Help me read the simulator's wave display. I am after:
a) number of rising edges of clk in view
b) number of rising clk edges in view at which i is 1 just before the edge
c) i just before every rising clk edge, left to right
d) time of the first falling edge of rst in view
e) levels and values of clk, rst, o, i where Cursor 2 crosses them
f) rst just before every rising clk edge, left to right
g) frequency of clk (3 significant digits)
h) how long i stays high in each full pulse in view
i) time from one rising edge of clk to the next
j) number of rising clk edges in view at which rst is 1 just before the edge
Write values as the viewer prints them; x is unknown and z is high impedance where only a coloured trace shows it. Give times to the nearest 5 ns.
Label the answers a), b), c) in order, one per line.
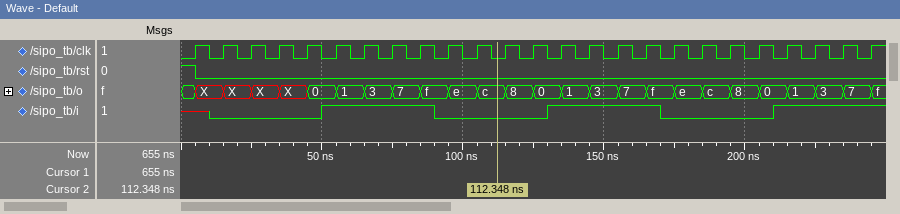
a) 25
b) 12
c) x 0 0 0 0 1 1 1 1 0 0 0 0 1 1 1 1 0 0 0 0 1 1 1 1
d) 5 ns
e) clk=0, rst=0, o=c, i=0
f) 1 0 0 0 0 0 0 0 0 0 0 0 0 0 0 0 0 0 0 0 0 0 0 0 0
g) 100 MHz
h) 40 ns, 40 ns
i) 10 ns
j) 1
